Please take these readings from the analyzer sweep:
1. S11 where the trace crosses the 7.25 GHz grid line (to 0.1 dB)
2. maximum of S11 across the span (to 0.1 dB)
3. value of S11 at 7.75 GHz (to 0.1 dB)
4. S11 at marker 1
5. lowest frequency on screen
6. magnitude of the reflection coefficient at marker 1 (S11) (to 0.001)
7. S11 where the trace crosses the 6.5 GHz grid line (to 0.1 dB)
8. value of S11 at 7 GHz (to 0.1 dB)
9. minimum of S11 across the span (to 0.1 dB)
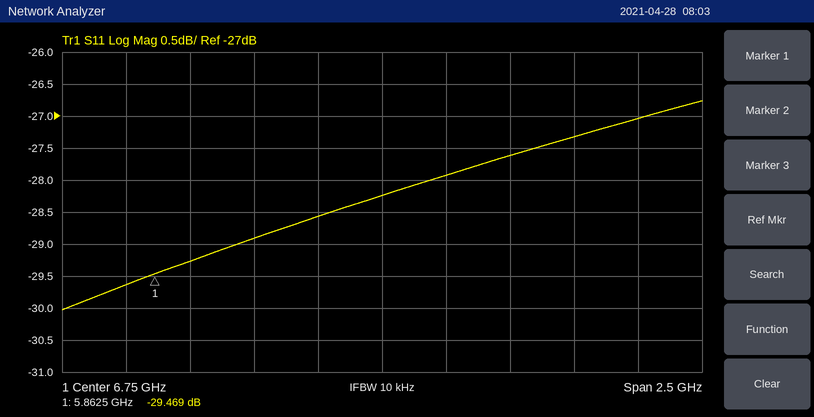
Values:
-27.6 dB
-26.8 dB
-27.0 dB
-29.469 dB
5.5 GHz
0.034
-28.6 dB
-27.9 dB
-30.0 dB
